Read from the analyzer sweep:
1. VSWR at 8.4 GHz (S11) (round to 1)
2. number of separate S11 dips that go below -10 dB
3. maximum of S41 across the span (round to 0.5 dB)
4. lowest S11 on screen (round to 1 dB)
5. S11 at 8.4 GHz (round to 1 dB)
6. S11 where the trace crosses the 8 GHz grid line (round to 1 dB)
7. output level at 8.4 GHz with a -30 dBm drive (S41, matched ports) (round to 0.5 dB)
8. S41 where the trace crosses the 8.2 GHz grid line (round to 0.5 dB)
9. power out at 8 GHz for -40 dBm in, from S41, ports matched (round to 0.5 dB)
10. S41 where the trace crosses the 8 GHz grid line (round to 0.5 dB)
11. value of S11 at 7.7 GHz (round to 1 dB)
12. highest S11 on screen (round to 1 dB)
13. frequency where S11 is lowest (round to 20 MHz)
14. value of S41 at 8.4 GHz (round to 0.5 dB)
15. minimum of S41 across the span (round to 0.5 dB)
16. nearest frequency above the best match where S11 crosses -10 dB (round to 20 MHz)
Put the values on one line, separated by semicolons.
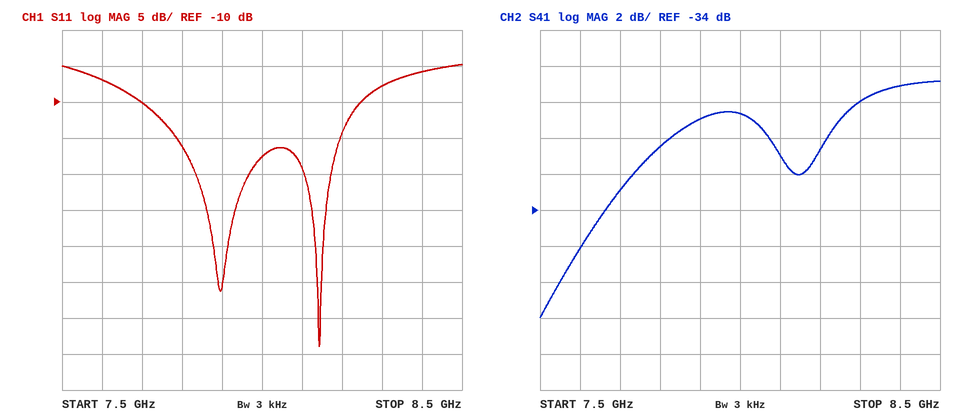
3; 2; -27.0 dB; -44 dB; -6 dB; -18 dB; -57.0 dBm; -30.5 dB; -68.5 dBm; -28.5 dB; -10 dB; -5 dB; 8.14 GHz; -27.0 dB; -40.0 dB; 8.24 GHz
